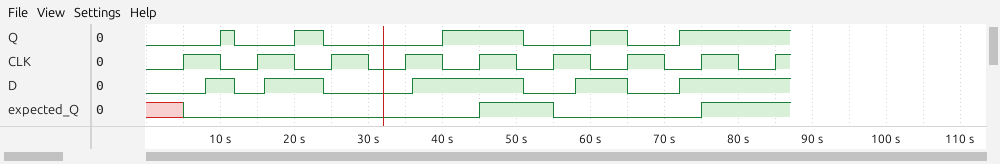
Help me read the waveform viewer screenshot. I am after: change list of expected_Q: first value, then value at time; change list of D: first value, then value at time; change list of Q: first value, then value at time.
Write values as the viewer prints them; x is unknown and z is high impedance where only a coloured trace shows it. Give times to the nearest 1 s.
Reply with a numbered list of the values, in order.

1. x, 0 at 5 s, 1 at 45 s, 0 at 55 s, 1 at 75 s
2. 0, 1 at 8 s, 0 at 12 s, 1 at 16 s, 0 at 24 s, 1 at 36 s, 0 at 51 s, 1 at 58 s, 0 at 65 s, 1 at 72 s
3. 0, 1 at 10 s, 0 at 12 s, 1 at 20 s, 0 at 24 s, 1 at 40 s, 0 at 51 s, 1 at 60 s, 0 at 65 s, 1 at 72 s
